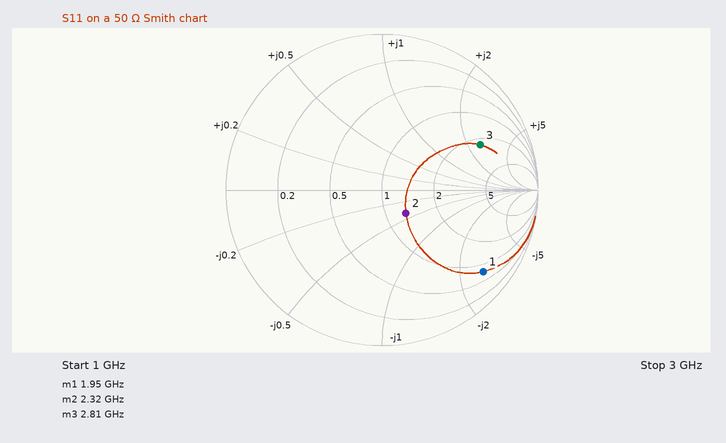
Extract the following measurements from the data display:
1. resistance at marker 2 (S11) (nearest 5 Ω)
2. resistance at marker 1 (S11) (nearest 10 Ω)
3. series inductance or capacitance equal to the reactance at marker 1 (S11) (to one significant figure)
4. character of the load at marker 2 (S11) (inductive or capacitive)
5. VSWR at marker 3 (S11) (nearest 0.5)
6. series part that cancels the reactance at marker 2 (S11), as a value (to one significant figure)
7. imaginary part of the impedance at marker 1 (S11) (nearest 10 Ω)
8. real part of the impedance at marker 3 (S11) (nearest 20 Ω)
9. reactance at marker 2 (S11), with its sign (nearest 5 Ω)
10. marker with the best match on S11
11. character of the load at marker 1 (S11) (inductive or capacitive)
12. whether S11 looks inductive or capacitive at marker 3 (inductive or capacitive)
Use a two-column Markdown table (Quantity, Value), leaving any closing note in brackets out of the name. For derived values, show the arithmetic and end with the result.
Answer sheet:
| Quantity | Value |
|---|---|
| resistance at marker 2 (S11) | 65 Ω |
| resistance at marker 1 (S11) | 40 Ω |
| series inductance or capacitance equal to the reactance at marker 1 (S11) | C = 1/(2π × 1.95 GHz × 130 Ω) ≈ 628 fF, so 600 fF to one significant figure |
| character of the load at marker 2 (S11) | capacitive |
| VSWR at marker 3 (S11) | 5.5 |
| series part that cancels the reactance at marker 2 (S11), as a value | L = 20 Ω/(2π × 2.32 GHz) ≈ 1 nH |
| imaginary part of the impedance at marker 1 (S11) | -130 Ω |
| real part of the impedance at marker 3 (S11) | 120 Ω |
| reactance at marker 2 (S11), with its sign | -20 Ω |
| marker with the best match on S11 | marker 2 |
| character of the load at marker 1 (S11) | capacitive |
| whether S11 looks inductive or capacitive at marker 3 | inductive |
